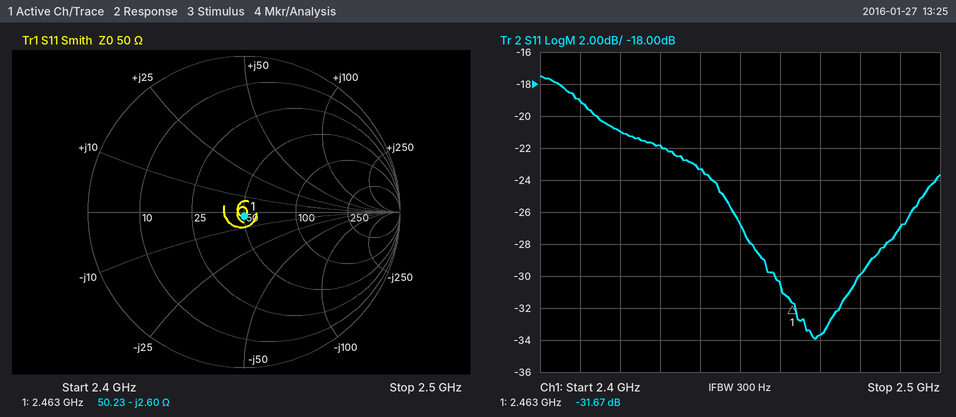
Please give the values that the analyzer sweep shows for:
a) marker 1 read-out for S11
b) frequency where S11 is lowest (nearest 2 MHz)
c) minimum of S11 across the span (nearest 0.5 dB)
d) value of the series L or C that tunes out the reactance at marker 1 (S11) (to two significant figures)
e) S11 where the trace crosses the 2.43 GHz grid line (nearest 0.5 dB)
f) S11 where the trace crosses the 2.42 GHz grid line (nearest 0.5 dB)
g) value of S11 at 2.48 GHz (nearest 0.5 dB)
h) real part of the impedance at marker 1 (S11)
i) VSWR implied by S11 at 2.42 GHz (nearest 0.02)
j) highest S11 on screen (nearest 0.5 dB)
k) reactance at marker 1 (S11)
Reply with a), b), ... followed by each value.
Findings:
a) -31.67 dB
b) 2.468 GHz
c) -34.0 dB
d) 170 pH
e) -22.0 dB
f) -21.0 dB
g) -30.0 dB
h) 50.23 Ω
i) 1.20
j) -17.5 dB
k) -2.60 Ω
